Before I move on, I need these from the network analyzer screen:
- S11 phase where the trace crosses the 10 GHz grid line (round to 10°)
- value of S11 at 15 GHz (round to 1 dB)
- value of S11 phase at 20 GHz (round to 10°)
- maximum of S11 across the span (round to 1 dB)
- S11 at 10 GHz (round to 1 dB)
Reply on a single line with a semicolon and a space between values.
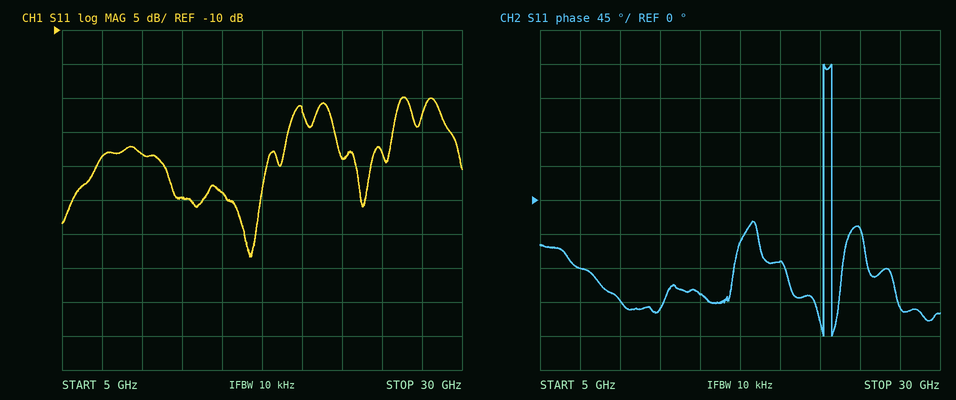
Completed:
-130°; -34 dB; -80°; -20 dB; -28 dB
